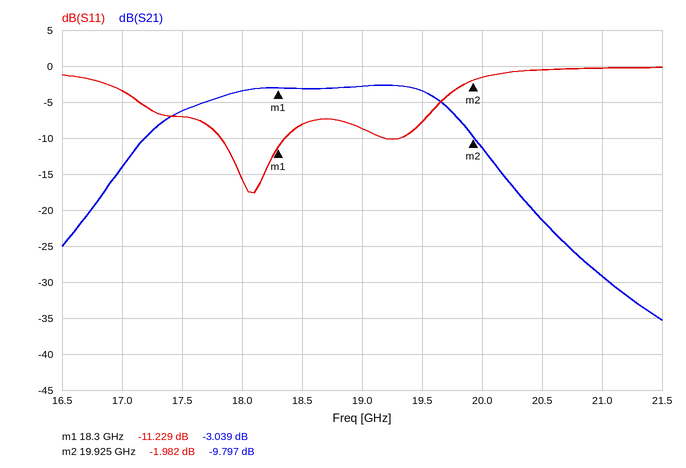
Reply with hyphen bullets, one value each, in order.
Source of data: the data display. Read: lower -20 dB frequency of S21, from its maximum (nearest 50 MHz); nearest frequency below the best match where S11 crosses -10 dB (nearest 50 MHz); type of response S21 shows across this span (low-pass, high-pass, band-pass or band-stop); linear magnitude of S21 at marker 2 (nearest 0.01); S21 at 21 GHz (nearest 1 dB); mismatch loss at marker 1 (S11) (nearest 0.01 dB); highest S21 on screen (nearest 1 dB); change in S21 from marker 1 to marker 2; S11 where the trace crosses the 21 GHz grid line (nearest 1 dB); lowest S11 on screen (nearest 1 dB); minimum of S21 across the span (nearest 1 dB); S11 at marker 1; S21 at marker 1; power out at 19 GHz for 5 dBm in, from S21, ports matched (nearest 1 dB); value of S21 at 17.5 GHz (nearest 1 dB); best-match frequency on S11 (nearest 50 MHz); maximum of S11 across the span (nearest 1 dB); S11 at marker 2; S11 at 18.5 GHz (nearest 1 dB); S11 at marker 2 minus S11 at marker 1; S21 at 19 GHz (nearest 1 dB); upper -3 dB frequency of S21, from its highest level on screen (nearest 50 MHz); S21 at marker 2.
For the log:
- 16.60 GHz
- 17.80 GHz
- band-pass
- 0.32
- -29 dB
- 0.34 dB
- -3 dB
- -6.758 dB
- 0 dB
- -18 dB
- -35 dB
- -11.229 dB
- -3.039 dB
- 2 dBm
- -6 dB
- 18.10 GHz
- 0 dB
- -1.982 dB
- -8 dB
- 9.247 dB
- -3 dB
- 19.70 GHz
- -9.797 dB
